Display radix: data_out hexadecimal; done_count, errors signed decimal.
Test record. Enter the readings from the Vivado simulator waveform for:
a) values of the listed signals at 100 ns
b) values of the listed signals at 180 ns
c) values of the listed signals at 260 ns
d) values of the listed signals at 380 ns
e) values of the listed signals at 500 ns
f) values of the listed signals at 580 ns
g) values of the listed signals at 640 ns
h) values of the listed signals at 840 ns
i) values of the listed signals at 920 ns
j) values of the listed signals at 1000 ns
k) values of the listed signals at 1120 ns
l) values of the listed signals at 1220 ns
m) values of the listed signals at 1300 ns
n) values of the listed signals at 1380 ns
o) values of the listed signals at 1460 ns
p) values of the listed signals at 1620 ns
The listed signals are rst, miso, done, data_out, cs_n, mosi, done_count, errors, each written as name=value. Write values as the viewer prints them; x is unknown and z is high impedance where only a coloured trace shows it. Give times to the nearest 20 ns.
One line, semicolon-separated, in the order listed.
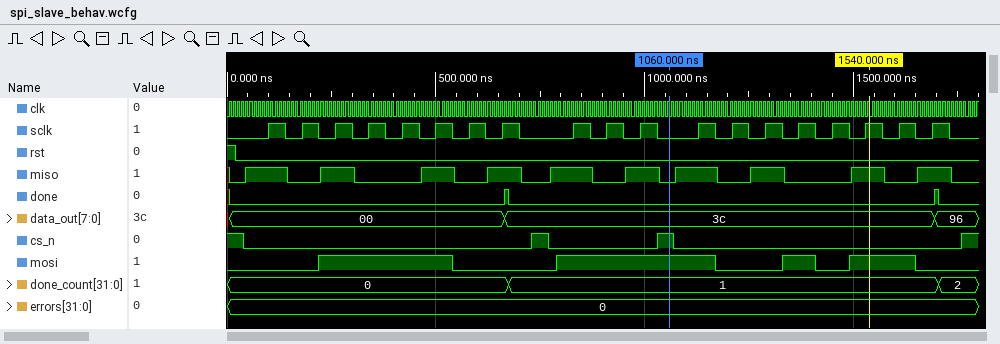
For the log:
rst=0, miso=1, done=0, data_out=00, cs_n=0, mosi=0, done_count=0, errors=0; rst=0, miso=0, done=0, data_out=00, cs_n=0, mosi=0, done_count=0, errors=0; rst=0, miso=1, done=0, data_out=00, cs_n=0, mosi=1, done_count=0, errors=0; rst=0, miso=0, done=0, data_out=00, cs_n=0, mosi=1, done_count=0, errors=0; rst=0, miso=1, done=0, data_out=00, cs_n=0, mosi=1, done_count=0, errors=0; rst=0, miso=0, done=0, data_out=00, cs_n=0, mosi=0, done_count=0, errors=0; rst=0, miso=1, done=0, data_out=00, cs_n=0, mosi=0, done_count=0, errors=0; rst=0, miso=1, done=0, data_out=3c, cs_n=0, mosi=1, done_count=1, errors=0; rst=0, miso=0, done=0, data_out=3c, cs_n=0, mosi=1, done_count=1, errors=0; rst=0, miso=1, done=0, data_out=3c, cs_n=0, mosi=1, done_count=1, errors=0; rst=0, miso=1, done=0, data_out=3c, cs_n=0, mosi=1, done_count=1, errors=0; rst=0, miso=0, done=0, data_out=3c, cs_n=0, mosi=0, done_count=1, errors=0; rst=0, miso=1, done=0, data_out=3c, cs_n=0, mosi=0, done_count=1, errors=0; rst=0, miso=0, done=0, data_out=3c, cs_n=0, mosi=1, done_count=1, errors=0; rst=0, miso=0, done=0, data_out=3c, cs_n=0, mosi=0, done_count=1, errors=0; rst=0, miso=0, done=0, data_out=3c, cs_n=0, mosi=1, done_count=1, errors=0
